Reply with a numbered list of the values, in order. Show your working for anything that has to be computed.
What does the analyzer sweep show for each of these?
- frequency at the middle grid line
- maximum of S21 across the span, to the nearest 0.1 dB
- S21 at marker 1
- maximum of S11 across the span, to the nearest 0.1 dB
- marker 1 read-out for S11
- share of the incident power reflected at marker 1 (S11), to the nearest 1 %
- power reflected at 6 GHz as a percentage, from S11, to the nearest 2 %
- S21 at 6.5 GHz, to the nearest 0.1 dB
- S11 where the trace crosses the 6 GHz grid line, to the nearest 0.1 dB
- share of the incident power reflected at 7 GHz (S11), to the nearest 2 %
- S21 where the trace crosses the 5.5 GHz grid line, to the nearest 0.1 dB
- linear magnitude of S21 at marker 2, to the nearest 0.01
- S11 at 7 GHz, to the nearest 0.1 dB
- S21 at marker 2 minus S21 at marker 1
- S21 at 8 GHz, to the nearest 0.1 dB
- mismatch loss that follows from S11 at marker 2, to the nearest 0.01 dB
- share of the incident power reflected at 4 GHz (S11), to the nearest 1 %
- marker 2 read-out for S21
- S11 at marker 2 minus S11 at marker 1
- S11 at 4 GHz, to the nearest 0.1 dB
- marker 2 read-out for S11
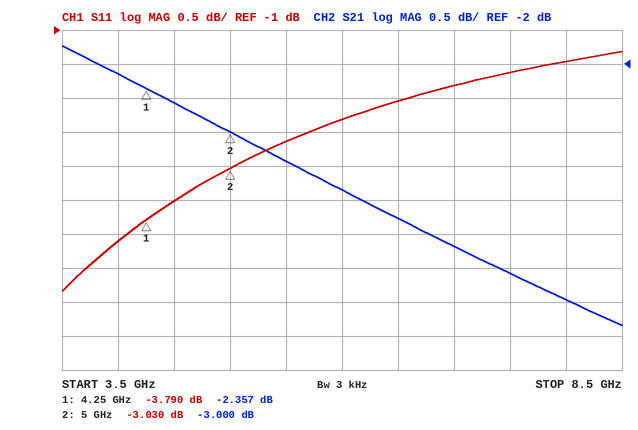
1. 6 GHz
2. -1.7 dB
3. -2.357 dB
4. -1.3 dB
5. -3.790 dB
6. 10^(-3.79/10) ≈ 42 %
7. 10^(-2.3/10) ≈ 58.9 %, so 58 % to the nearest 2 %
8. -4.3 dB
9. -2.3 dB
10. 10^(-1.8/10) ≈ 66 %
11. -3.4 dB
12. 10^(-3/20) ≈ 0.71
13. -1.8 dB
14. -3 − (-2.357) = -0.643 dB
15. -5.5 dB
16. −10 log10(1 − 10^(-3.03/10)) ≈ 2.99 dB
17. 10^(-4.1/10) ≈ 39 %
18. -3.000 dB
19. -3.03 − (-3.79) = 0.760 dB
20. -4.1 dB
21. -3.030 dB
